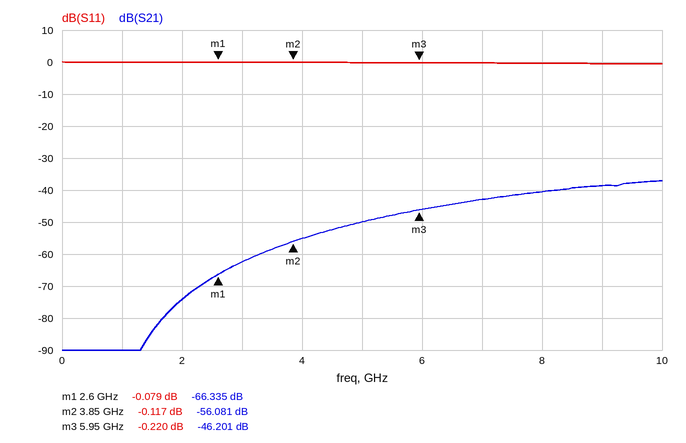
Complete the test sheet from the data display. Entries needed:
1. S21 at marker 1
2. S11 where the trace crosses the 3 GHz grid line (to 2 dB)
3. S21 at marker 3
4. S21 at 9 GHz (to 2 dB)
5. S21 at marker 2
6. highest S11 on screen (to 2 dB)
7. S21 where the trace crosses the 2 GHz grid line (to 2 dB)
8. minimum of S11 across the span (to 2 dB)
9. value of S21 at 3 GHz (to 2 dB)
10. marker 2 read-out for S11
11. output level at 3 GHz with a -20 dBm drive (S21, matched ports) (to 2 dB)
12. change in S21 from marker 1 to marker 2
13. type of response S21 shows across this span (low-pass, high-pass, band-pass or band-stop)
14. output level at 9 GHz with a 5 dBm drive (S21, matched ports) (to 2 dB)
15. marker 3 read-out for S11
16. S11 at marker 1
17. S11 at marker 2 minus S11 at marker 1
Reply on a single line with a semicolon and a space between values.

-66.335 dB; 0 dB; -46.201 dB; -38 dB; -56.081 dB; 0 dB; -74 dB; 0 dB; -62 dB; -0.117 dB; -82 dBm; 10.254 dB; high-pass; -34 dBm; -0.220 dB; -0.079 dB; -0.038 dB
